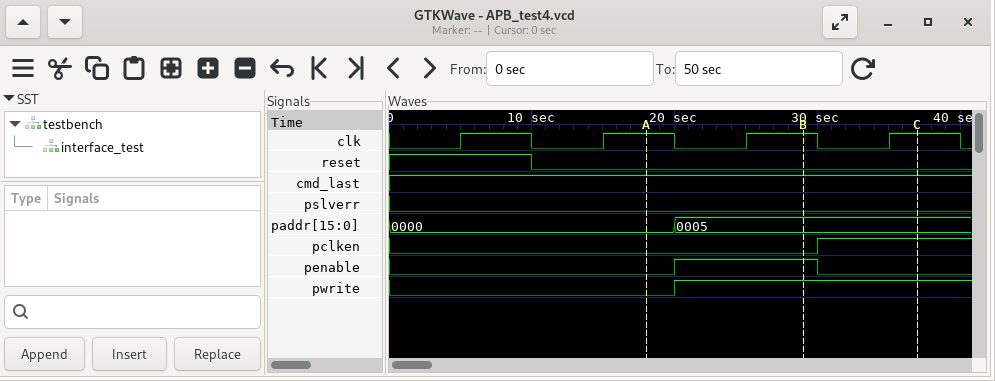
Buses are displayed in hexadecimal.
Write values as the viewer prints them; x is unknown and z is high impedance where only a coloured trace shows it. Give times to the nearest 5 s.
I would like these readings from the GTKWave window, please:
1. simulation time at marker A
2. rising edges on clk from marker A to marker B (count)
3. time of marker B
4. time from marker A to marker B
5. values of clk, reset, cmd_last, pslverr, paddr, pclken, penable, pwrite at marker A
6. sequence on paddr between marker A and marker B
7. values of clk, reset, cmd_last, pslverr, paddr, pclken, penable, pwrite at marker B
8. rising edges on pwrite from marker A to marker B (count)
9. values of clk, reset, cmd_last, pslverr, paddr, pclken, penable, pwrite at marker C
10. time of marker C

20 s
1
30 s
10 s
clk=1, reset=0, cmd_last=1, pslverr=0, paddr=0000, pclken=0, penable=0, pwrite=0
0000, 0005
clk=1, reset=0, cmd_last=1, pslverr=0, paddr=0005, pclken=0, penable=1, pwrite=1
1
clk=1, reset=0, cmd_last=1, pslverr=0, paddr=0005, pclken=1, penable=0, pwrite=1
35 s
